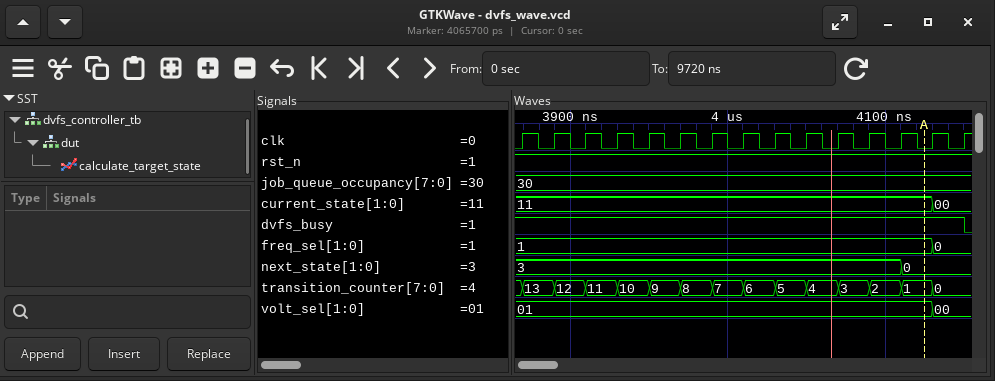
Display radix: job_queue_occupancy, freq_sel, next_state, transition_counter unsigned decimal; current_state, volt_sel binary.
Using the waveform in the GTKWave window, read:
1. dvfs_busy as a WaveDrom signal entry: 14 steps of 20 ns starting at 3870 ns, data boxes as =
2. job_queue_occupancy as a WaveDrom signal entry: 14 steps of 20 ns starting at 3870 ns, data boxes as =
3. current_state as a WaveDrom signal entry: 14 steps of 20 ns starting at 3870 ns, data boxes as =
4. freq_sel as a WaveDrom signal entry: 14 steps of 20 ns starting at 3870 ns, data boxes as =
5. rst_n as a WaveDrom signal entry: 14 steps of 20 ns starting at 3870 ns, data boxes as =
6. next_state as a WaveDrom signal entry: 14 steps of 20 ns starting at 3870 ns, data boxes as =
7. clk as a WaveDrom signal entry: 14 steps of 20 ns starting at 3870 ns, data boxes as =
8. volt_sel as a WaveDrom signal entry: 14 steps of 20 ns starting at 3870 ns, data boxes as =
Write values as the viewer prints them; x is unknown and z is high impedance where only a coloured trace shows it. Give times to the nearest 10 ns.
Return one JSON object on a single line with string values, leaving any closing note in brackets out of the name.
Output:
{"dvfs_busy as a WaveDrom signal entry: 14 steps of 20 ns starting at 3870 ns, data boxes as =": "{name: 'dvfs_busy', wave: '1.............'}", "job_queue_occupancy as a WaveDrom signal entry: 14 steps of 20 ns starting at 3870 ns, data boxes as =": "{name: 'job_queue_occupancy', wave: '=.............', data: '30'}", "current_state as a WaveDrom signal entry: 14 steps of 20 ns starting at 3870 ns, data boxes as =": "{name: 'current_state', wave: '=............=', data: '11 00'}", "freq_sel as a WaveDrom signal entry: 14 steps of 20 ns starting at 3870 ns, data boxes as =": "{name: 'freq_sel', wave: '=............=', data: '1 0'}", "rst_n as a WaveDrom signal entry: 14 steps of 20 ns starting at 3870 ns, data boxes as =": "{name: 'rst_n', wave: '1.............'}", "next_state as a WaveDrom signal entry: 14 steps of 20 ns starting at 3870 ns, data boxes as =": "{name: 'next_state', wave: '=...........=.', data: '3 0'}", "clk as a WaveDrom signal entry: 14 steps of 20 ns starting at 3870 ns, data boxes as =": "{name: 'clk', wave: 'p.............'}", "volt_sel as a WaveDrom signal entry: 14 steps of 20 ns starting at 3870 ns, data boxes as =": "{name: 'volt_sel', wave: '=............=', data: '01 00'}"}
